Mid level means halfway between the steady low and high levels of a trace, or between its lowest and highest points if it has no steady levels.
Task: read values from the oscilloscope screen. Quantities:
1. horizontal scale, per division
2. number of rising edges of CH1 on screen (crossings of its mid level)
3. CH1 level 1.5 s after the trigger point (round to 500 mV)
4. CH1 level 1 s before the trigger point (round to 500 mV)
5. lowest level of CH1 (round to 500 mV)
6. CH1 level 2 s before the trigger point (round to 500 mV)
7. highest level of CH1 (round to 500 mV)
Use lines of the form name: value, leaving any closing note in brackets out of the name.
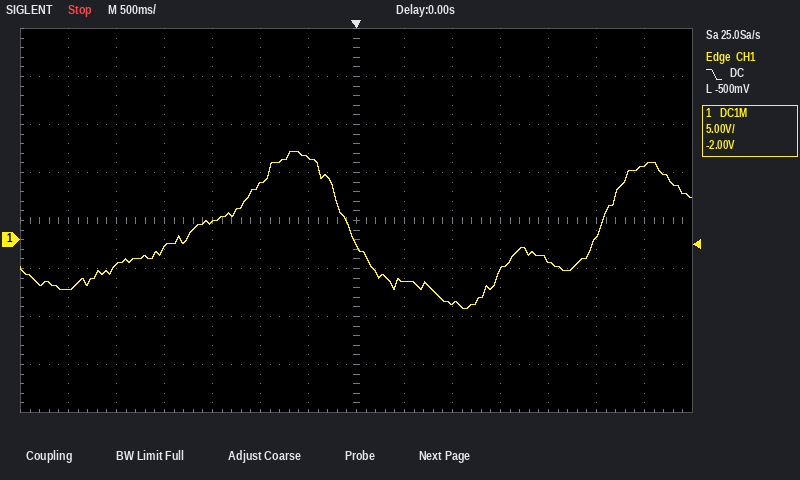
horizontal scale, per division: 500 ms
number of rising edges of CH1 on screen: 2
CH1 level 1.5 s after the trigger point: -3.0 V
CH1 level 1 s before the trigger point: 6.0 V
lowest level of CH1: -7.0 V
CH1 level 2 s before the trigger point: -1.0 V
highest level of CH1: 9.0 V
